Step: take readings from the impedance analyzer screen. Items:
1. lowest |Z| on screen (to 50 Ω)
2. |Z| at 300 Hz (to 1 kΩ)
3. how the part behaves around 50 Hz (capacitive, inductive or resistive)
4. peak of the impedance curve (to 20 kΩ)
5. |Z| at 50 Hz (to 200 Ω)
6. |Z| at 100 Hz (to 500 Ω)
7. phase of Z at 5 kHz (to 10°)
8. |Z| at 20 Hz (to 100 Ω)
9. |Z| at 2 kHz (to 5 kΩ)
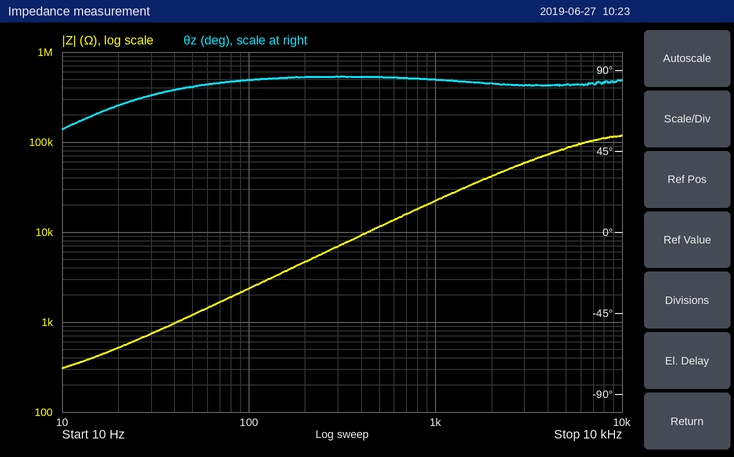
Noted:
300 Ω
7 kΩ
inductive
120 kΩ
1.2 kΩ
2.5 kΩ
80°
500 Ω
40 kΩ
